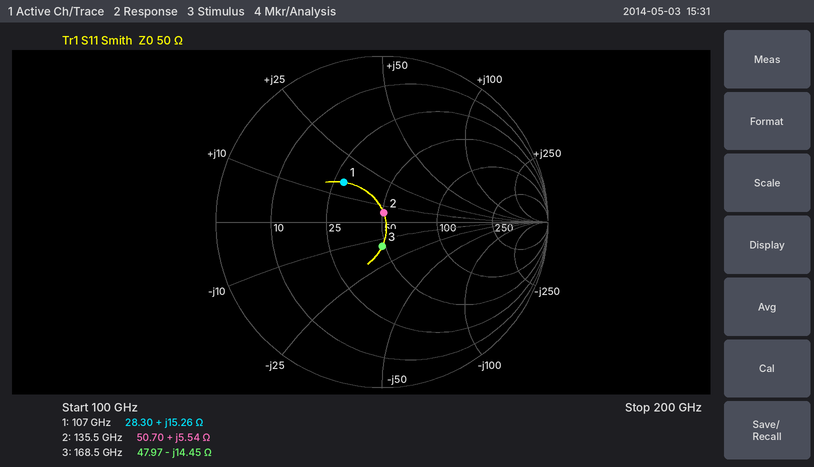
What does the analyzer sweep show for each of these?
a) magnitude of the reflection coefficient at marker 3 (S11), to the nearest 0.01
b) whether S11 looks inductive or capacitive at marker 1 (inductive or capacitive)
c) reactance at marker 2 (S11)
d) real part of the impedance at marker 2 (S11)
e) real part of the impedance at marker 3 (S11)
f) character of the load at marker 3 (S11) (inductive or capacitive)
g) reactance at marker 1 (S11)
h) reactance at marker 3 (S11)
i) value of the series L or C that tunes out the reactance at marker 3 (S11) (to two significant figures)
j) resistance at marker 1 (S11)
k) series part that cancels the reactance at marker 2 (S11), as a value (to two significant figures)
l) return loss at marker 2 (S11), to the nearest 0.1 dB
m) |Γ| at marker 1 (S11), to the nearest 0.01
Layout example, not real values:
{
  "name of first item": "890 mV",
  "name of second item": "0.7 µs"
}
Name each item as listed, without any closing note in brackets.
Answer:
{
  "magnitude of the reflection coefficient at marker 3 (S11), to the nearest 0.01": "0.15",
  "whether S11 looks inductive or capacitive at marker 1": "inductive",
  "reactance at marker 2": "+5.54 Ω",
  "real part of the impedance at marker 2": "50.70 Ω",
  "real part of the impedance at marker 3": "47.97 Ω",
  "character of the load at marker 3 (S11)": "capacitive",
  "reactance at marker 1": "+15.26 Ω",
  "reactance at marker 3": "-14.45 Ω",
  "value of the series L or C that tunes out the reactance at marker 3 (S11)": "14 pH",
  "resistance at marker 1": "28.30 Ω",
  "series part that cancels the reactance at marker 2 (S11), as a value": "210 fF",
  "return loss at marker 2 (S11), to the nearest 0.1 dB": "25.1 dB",
  "|Γ| at marker 1 (S11), to the nearest 0.01": "0.33"
}
